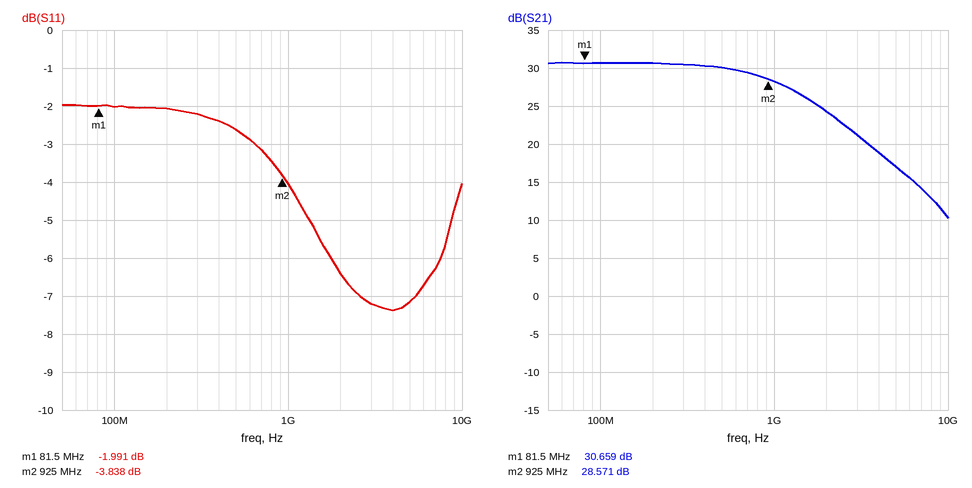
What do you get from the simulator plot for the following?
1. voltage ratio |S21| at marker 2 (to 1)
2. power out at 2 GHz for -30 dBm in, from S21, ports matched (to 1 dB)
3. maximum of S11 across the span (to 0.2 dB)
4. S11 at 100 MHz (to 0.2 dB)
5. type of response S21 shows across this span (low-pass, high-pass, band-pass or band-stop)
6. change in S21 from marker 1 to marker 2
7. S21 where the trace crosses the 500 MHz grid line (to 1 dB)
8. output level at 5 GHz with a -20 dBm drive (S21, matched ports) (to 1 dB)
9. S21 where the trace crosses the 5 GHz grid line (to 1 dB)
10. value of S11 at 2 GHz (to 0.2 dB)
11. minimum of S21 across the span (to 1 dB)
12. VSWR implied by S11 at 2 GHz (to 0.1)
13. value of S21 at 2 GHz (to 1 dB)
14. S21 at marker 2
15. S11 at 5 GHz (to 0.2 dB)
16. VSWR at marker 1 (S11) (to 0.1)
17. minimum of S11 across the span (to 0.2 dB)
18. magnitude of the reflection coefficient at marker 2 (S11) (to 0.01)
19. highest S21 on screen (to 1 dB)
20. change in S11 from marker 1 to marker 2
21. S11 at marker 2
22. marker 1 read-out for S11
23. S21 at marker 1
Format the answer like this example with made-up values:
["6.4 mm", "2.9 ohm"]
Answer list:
["27", "-6 dBm", "-2.0 dB", "-2.0 dB", "low-pass", "-2.088 dB", "30 dB", "-3 dBm", "17 dB", "-6.4 dB", "10 dB", "2.8", "24 dB", "28.571 dB", "-7.2 dB", "8.8", "-7.4 dB", "0.64", "31 dB", "-1.847 dB", "-3.838 dB", "-1.991 dB", "30.659 dB"]
